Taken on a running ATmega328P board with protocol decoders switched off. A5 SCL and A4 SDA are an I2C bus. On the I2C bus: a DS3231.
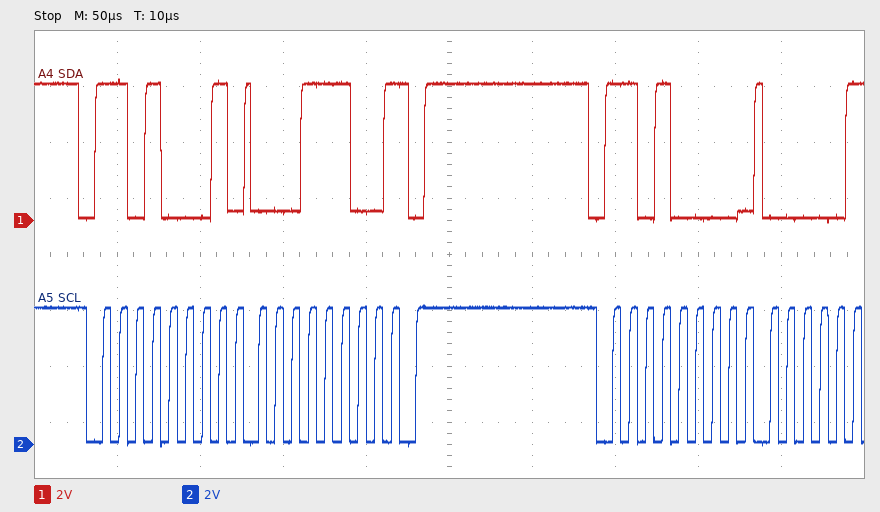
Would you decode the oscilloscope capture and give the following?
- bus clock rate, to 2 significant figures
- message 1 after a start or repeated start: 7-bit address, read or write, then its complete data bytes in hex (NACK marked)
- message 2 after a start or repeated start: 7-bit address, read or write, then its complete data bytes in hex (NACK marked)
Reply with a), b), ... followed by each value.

a) 100 kHz
b) 0x68 read: 1C NACK
c) 0x68 write
